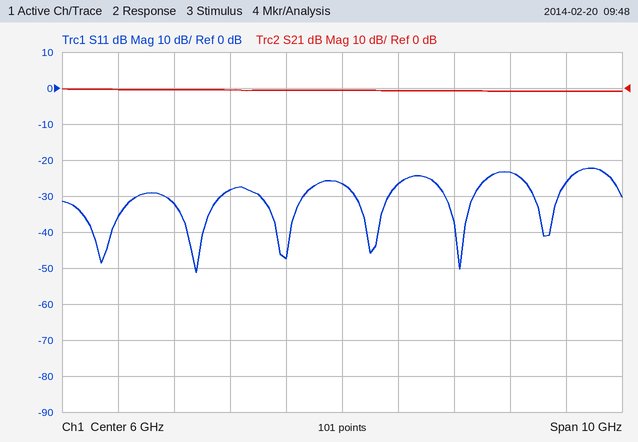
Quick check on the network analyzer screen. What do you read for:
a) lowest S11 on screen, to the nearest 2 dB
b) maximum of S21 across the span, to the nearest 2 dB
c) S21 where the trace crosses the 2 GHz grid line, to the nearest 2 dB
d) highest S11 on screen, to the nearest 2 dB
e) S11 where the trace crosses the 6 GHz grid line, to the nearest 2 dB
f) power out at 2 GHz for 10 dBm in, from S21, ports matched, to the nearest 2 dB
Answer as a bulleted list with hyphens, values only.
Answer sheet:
- -52 dB
- 0 dB
- 0 dB
- -22 dB
- -26 dB
- 10 dBm
